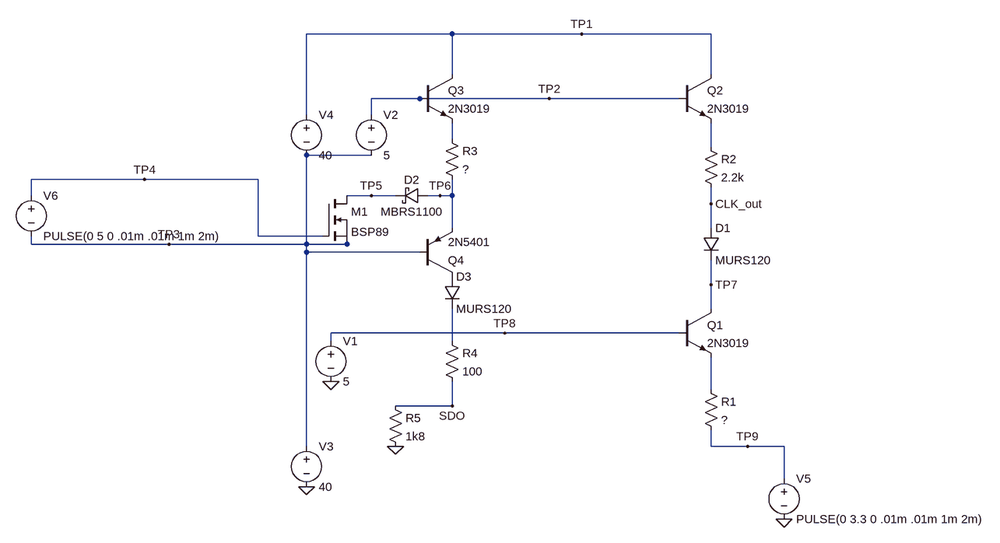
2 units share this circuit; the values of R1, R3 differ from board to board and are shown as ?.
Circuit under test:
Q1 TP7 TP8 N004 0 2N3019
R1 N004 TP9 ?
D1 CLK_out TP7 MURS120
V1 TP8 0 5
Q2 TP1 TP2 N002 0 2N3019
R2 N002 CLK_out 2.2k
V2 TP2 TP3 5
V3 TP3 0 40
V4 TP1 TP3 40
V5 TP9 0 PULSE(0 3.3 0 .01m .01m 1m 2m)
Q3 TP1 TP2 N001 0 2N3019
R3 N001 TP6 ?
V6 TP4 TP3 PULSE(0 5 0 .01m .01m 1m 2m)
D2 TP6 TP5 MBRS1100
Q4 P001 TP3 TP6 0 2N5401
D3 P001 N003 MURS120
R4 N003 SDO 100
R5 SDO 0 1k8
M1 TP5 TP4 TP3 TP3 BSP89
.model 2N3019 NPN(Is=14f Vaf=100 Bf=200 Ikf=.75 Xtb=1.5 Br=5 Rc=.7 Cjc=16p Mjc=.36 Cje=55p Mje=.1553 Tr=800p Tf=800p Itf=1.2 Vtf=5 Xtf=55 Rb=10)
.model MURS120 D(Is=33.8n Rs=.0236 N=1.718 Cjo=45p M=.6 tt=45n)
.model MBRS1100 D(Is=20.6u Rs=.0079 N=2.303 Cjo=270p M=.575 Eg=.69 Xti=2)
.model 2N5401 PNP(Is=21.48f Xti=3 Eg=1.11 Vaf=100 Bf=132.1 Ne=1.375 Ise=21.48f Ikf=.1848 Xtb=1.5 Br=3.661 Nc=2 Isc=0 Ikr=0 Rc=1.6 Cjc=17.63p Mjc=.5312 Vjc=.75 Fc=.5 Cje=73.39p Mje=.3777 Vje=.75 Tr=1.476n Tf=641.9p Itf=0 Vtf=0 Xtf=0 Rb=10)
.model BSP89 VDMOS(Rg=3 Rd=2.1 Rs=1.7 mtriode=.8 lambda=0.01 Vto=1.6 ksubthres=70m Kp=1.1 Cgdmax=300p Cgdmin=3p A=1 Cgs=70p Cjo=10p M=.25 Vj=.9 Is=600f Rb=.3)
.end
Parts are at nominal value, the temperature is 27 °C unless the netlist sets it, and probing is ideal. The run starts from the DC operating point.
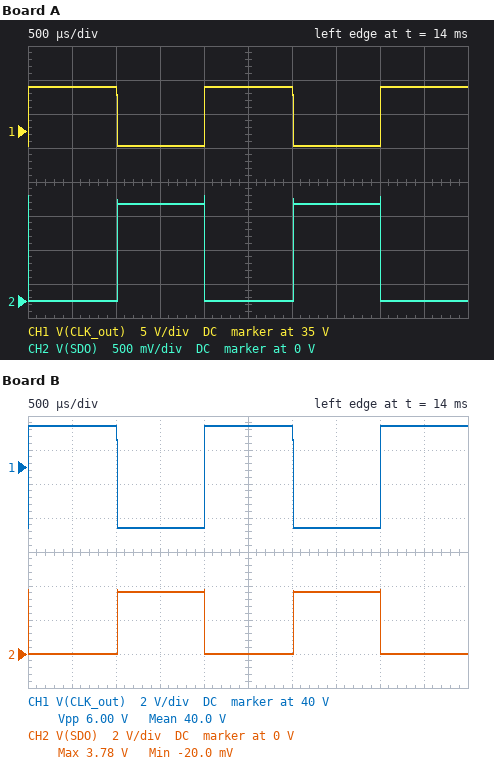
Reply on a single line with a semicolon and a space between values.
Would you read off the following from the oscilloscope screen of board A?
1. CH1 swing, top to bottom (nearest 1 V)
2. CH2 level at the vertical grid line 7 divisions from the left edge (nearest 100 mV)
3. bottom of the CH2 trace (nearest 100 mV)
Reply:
9 V; 1.4 V; 0 V
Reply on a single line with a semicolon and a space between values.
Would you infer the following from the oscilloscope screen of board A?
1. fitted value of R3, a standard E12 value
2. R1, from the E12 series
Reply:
4.7 kΩ; 820 Ω
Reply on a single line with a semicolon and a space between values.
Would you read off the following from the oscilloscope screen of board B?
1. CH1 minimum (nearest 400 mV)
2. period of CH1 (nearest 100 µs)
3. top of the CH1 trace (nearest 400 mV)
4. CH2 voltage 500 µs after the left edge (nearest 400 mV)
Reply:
36.4 V; 2.0 ms; 42.4 V; 0 V
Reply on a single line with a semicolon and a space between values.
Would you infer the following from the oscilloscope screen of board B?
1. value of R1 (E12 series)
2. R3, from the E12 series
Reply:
1.2 kΩ; 1.8 kΩ
